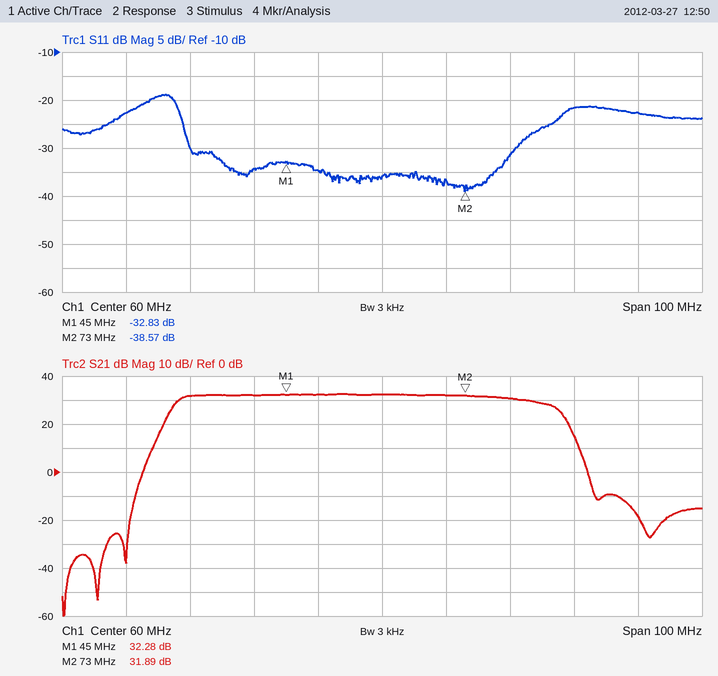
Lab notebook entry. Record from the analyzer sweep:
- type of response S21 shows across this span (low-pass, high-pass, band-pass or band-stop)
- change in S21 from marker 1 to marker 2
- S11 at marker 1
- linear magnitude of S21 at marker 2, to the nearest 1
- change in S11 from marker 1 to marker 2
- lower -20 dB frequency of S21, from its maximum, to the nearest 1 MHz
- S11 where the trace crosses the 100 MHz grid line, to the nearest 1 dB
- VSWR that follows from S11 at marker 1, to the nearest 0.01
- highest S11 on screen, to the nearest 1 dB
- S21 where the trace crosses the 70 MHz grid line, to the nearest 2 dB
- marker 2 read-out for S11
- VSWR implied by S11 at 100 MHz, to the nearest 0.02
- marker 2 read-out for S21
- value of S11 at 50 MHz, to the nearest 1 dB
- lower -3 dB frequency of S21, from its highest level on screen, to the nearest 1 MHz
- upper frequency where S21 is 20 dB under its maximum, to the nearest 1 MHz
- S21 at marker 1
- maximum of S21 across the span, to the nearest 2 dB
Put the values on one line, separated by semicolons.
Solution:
band-pass; -0.39 dB; -32.83 dB; 39; -5.74 dB; 25 MHz; -23 dB; 1.05; -19 dB; 32 dB; -38.57 dB; 1.16; 31.89 dB; -35 dB; 28 MHz; 90 MHz; 32.28 dB; 32 dB
